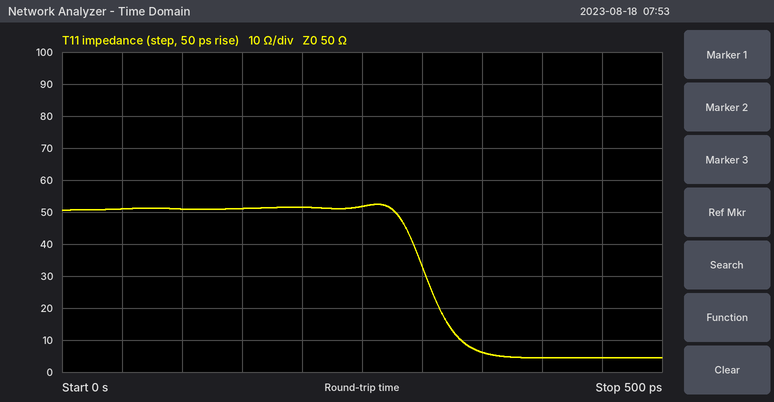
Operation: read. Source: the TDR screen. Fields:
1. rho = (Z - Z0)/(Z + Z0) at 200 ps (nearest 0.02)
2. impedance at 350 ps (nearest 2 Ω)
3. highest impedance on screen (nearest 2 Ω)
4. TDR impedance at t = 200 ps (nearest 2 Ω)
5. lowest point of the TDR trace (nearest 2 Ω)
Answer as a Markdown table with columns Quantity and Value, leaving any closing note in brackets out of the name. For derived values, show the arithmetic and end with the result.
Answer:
| Quantity | Value |
|---|---|
| rho = (Z - Z0)/(Z + Z0) at 200 ps | (52 − 50)/(52 + 50) ≈ +0.02 |
| impedance at 350 ps | 6 Ω |
| highest impedance on screen | 52 Ω |
| TDR impedance at t = 200 ps | 52 Ω |
| lowest point of the TDR trace | 4 Ω |
